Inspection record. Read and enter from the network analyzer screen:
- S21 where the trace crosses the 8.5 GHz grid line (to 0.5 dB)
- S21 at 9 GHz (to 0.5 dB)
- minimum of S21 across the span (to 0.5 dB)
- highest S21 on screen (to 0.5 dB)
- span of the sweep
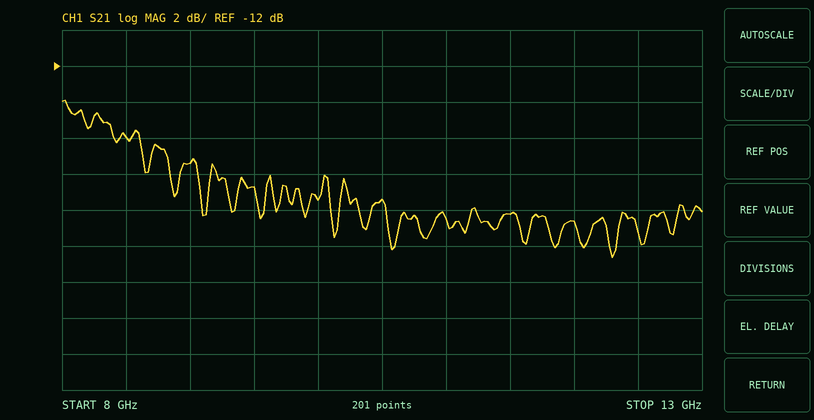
-16.0 dB
-17.5 dB
-22.5 dB
-14.0 dB
5 GHz
